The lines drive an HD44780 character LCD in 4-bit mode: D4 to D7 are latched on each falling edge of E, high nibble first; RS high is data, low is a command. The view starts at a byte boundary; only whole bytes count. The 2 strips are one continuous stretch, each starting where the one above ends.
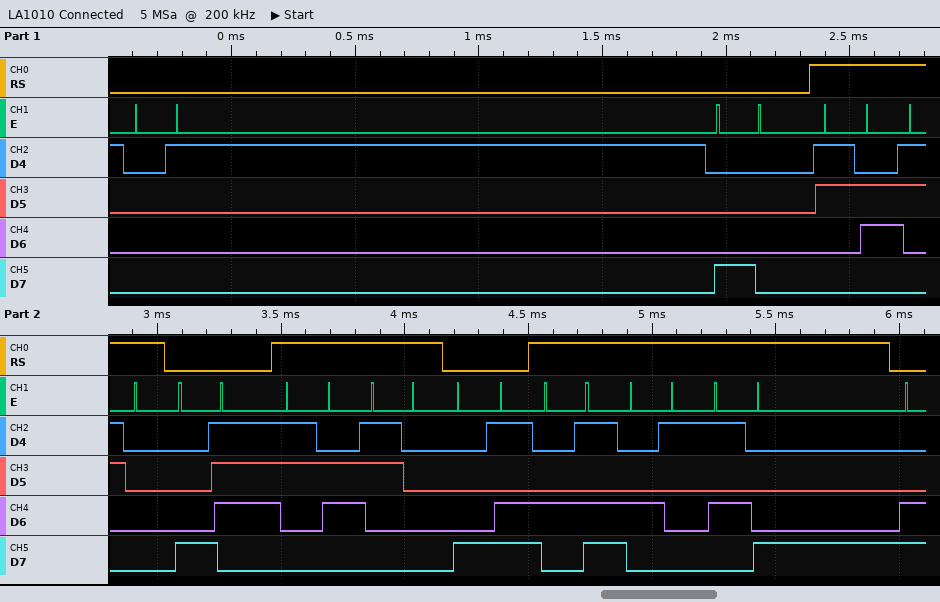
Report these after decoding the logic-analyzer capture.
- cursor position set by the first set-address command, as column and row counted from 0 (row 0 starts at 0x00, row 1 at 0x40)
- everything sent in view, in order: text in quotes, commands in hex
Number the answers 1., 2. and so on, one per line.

1. column 0, row 0
2. 0x01 0x80 "60" 0x87 "60" 0x8D "MAX"
